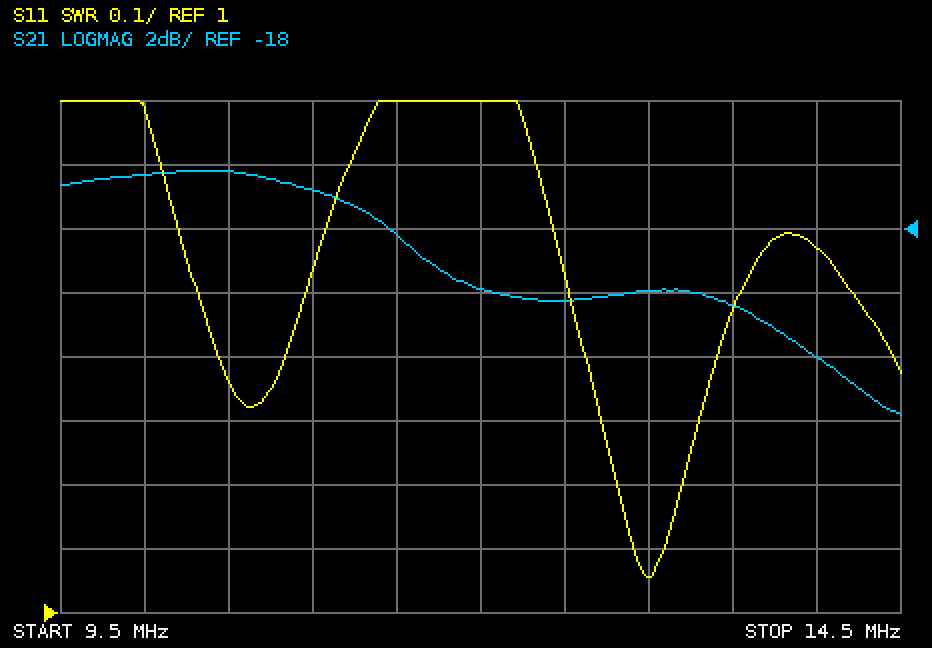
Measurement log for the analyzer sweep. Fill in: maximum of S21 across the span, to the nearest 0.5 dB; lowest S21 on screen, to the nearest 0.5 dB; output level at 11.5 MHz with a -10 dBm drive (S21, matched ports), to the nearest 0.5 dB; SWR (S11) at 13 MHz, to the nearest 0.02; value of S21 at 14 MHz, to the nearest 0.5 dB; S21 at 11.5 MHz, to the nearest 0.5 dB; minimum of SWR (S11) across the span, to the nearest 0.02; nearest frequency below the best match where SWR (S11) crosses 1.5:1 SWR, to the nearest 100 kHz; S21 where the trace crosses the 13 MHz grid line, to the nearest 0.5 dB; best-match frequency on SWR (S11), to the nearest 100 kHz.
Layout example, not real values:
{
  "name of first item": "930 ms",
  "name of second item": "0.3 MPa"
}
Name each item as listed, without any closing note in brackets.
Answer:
{
  "maximum of S21 across the span, to the nearest 0.5 dB": "-16.0 dB",
  "lowest S21 on screen, to the nearest 0.5 dB": "-24.0 dB",
  "output level at 11.5 MHz with a -10 dBm drive (S21, matched ports), to the nearest 0.5 dB": "-28.0 dBm",
  "SWR (S11) at 13 MHz, to the nearest 0.02": "1.06",
  "value of S21 at 14 MHz, to the nearest 0.5 dB": "-22.0 dB",
  "S21 at 11.5 MHz, to the nearest 0.5 dB": "-18.0 dB",
  "minimum of SWR (S11) across the span, to the nearest 0.02": "1.06",
  "nearest frequency below the best match where SWR (S11) crosses 1.5:1 SWR, to the nearest 100 kHz": "12.5 MHz",
  "S21 where the trace crosses the 13 MHz grid line, to the nearest 0.5 dB": "-20.0 dB",
  "best-match frequency on SWR (S11), to the nearest 100 kHz": "13.0 MHz"
}
